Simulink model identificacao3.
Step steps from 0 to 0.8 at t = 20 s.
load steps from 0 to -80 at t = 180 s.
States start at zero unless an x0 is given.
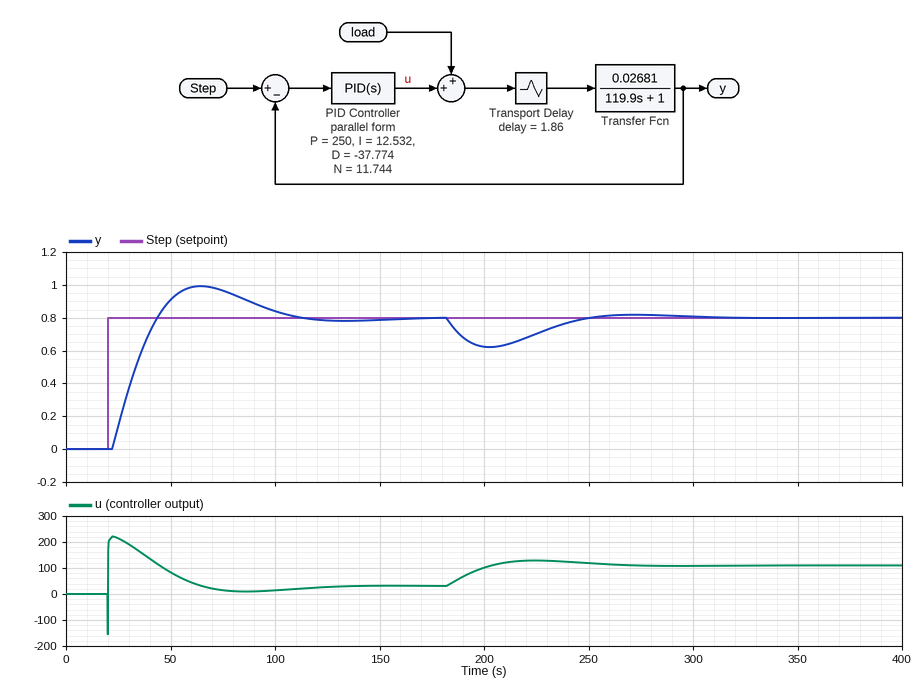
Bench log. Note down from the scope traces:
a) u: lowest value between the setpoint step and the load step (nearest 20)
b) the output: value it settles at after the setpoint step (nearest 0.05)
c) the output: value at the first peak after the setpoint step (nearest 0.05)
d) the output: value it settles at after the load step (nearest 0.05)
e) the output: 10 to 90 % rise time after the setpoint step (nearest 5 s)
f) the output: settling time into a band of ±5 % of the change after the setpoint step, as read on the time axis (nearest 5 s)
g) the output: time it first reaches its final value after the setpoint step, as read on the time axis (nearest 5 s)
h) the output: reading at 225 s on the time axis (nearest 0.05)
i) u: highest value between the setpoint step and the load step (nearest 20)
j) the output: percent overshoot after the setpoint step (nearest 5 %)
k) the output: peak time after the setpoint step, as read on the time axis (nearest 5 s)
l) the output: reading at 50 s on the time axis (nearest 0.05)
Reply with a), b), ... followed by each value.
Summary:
a) -160
b) 0.80
c) 1.00
d) 0.80
e) 15 s
f) 100 s
g) 45 s
h) 0.70
i) 220
j) 25 %
k) 65 s
l) 0.90
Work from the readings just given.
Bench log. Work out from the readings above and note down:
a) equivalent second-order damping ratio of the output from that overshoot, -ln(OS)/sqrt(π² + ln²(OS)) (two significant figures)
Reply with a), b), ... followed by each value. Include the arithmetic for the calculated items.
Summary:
a) ln(0.25) = -1.386; 1.386 / sqrt(9.870 + 1.922) = 0.40
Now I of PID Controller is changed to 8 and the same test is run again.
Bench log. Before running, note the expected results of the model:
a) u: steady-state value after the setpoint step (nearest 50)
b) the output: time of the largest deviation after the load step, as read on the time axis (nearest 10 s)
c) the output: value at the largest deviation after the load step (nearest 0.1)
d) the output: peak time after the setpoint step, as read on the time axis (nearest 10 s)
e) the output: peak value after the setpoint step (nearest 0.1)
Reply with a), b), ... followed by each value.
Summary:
a) 50
b) 210 s
c) 0.6
d) 70 s
e) 0.9
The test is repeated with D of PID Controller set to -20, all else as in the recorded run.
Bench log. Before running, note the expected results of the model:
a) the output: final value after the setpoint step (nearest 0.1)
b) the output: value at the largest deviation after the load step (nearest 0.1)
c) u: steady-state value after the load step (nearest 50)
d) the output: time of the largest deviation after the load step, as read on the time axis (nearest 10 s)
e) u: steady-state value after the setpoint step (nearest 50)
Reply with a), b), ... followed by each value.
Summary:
a) 0.8
b) 0.6
c) 100
d) 200 s
e) 50
